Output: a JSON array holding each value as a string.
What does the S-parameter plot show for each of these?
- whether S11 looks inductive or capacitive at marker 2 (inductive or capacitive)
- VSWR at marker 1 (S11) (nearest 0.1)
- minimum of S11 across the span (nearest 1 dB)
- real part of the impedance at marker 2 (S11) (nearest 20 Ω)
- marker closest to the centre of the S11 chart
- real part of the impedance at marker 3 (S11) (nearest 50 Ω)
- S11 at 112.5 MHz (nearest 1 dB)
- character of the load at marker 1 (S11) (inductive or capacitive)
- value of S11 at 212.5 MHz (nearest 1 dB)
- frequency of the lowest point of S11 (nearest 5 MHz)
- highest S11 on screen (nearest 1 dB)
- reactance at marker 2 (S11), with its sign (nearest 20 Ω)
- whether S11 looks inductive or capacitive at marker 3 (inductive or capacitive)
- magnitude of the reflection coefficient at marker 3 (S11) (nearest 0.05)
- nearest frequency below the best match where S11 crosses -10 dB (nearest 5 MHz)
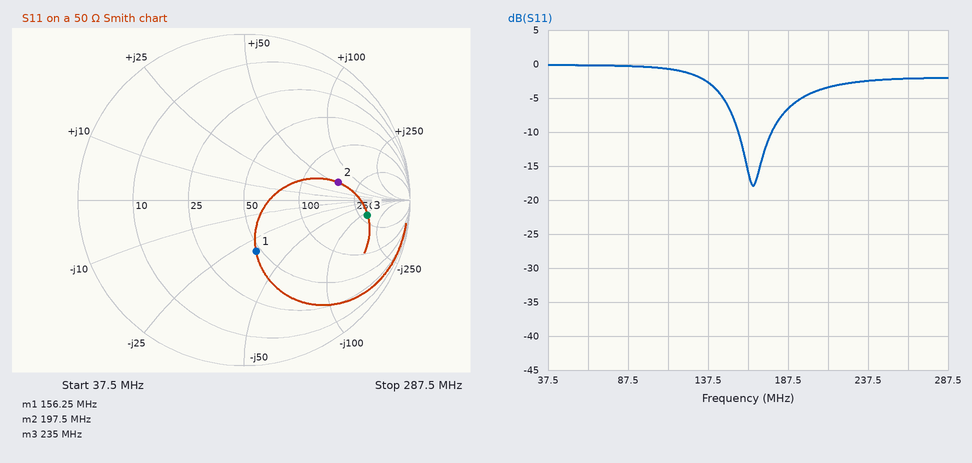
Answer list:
["inductive", "1.9", "-18 dB", "160 Ω", "marker 1", "300 Ω", "-1 dB", "capacitive", "-3 dB", "165 MHz", "0 dB", "+60 Ω", "capacitive", "0.75", "155 MHz"]
